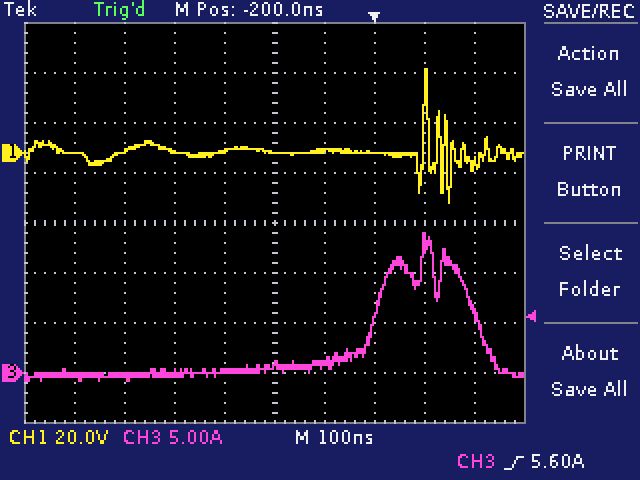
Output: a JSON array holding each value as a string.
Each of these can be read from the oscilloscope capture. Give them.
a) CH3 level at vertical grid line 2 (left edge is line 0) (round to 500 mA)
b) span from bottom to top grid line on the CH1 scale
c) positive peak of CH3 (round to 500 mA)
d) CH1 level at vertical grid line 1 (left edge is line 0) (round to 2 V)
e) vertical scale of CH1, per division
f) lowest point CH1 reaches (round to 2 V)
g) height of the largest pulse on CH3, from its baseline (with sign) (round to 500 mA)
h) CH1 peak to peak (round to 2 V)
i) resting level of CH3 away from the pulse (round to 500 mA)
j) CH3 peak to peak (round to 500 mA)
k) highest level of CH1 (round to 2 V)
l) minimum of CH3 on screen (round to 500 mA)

["-500 mA", "160 V", "14.0 A", "0 V", "20 V", "-20 V", "+14.0 A", "54 V", "0.0 A", "15.0 A", "34 V", "-1.0 A"]
